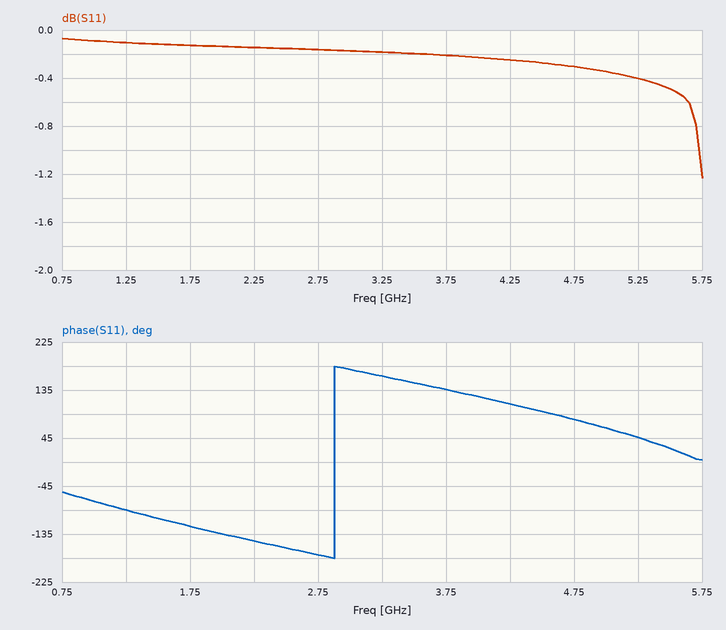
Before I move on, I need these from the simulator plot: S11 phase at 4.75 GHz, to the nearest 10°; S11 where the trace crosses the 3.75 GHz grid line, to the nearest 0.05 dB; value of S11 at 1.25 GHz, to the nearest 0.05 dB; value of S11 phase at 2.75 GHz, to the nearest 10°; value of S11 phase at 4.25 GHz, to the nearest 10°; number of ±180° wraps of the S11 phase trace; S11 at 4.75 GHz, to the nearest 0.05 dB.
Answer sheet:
80°
-0.20 dB
-0.10 dB
-170°
110°
1
-0.30 dB
